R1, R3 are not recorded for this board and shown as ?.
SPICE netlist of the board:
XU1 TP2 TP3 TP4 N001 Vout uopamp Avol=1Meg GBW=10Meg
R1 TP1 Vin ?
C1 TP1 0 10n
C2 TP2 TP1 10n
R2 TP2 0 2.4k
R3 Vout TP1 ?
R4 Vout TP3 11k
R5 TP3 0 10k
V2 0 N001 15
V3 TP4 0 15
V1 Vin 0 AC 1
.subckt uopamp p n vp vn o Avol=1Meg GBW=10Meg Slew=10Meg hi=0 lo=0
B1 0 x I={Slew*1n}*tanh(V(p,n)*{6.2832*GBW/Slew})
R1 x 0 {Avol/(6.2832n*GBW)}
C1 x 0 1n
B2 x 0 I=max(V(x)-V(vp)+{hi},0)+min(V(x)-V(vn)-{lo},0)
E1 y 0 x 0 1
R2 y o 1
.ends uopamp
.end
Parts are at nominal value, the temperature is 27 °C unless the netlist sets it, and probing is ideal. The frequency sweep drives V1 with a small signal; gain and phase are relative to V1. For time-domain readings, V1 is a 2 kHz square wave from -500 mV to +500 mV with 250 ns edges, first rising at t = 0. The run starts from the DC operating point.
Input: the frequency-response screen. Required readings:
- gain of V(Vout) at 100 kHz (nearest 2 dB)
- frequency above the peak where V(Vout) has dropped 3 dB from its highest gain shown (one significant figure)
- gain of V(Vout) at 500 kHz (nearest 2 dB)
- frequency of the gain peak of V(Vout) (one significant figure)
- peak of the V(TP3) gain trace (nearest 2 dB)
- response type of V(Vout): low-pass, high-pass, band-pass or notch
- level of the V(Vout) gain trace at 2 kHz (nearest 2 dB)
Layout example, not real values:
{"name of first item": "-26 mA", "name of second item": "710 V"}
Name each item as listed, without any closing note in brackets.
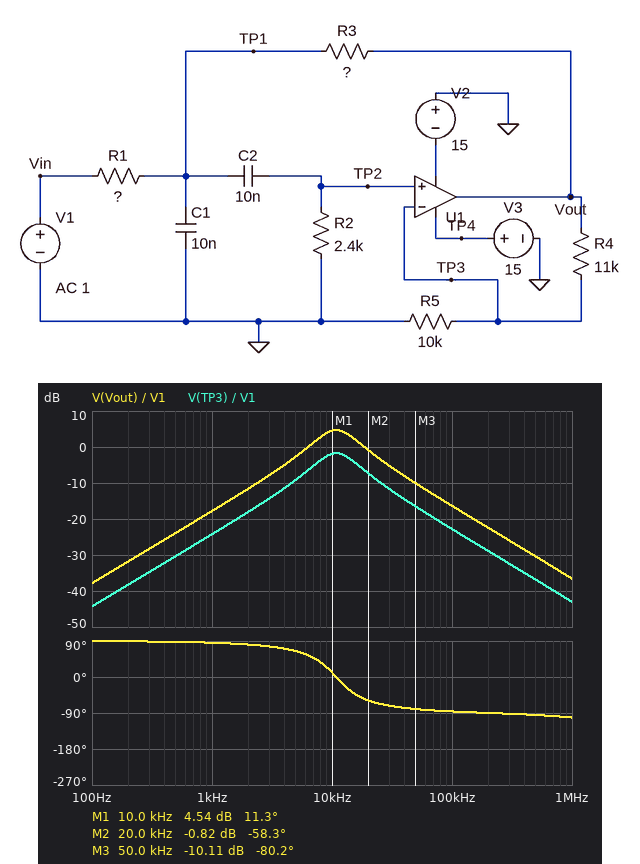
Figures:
{"gain of V(Vout) at 100 kHz": "-16 dB", "frequency above the peak where V(Vout) has dropped 3 dB from its highest gain shown": "20 kHz", "gain of V(Vout) at 500 kHz": "-30 dB", "frequency of the gain peak of V(Vout)": "10 kHz", "peak of the V(TP3) gain trace": "-2 dB", "response type of V(Vout): low-pass, high-pass, band-pass or notch": "band-pass", "level of the V(Vout) gain trace at 2 kHz": "-12 dB"}
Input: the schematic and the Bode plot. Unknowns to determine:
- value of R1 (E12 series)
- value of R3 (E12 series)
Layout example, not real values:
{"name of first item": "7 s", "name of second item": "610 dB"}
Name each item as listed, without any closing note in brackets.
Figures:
{"value of R1": "2.2 kΩ", "value of R3": "1.5 kΩ"}
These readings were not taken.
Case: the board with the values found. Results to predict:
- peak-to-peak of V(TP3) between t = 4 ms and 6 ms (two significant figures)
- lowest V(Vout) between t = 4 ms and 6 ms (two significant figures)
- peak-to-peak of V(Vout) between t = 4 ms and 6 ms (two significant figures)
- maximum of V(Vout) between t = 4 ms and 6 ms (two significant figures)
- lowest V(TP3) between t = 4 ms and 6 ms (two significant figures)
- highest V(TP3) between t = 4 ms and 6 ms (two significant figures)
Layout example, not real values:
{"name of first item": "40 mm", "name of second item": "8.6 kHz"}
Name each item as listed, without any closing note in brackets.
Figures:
{"peak-to-peak of V(TP3) between t = 4 ms and 6 ms": "800 mV", "lowest V(Vout) between t = 4 ms and 6 ms": "-840 mV", "peak-to-peak of V(Vout) between t = 4 ms and 6 ms": "1.7 V", "maximum of V(Vout) between t = 4 ms and 6 ms": "840 mV", "lowest V(TP3) between t = 4 ms and 6 ms": "-400 mV", "highest V(TP3) between t = 4 ms and 6 ms": "400 mV"}
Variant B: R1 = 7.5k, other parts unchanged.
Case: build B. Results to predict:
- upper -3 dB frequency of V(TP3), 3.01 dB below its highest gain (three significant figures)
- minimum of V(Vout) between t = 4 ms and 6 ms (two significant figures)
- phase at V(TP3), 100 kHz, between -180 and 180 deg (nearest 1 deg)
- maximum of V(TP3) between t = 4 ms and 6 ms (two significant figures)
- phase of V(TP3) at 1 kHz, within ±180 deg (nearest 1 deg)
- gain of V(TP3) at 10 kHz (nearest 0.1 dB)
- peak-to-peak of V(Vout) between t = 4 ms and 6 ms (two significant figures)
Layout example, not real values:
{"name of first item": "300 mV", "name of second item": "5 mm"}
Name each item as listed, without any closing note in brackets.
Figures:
{"upper -3 dB frequency of V(TP3), 3.01 dB below its highest gain": "11.2 kHz", "minimum of V(Vout) between t = 4 ms and 6 ms": "-360 mV", "phase at V(TP3), 100 kHz, between -180 and 180 deg": "-89 deg", "maximum of V(TP3) between t = 4 ms and 6 ms": "170 mV", "phase of V(TP3) at 1 kHz, within ±180 deg": "87 deg", "gain of V(TP3) at 10 kHz": "-5.6 dB", "peak-to-peak of V(Vout) between t = 4 ms and 6 ms": "720 mV"}
